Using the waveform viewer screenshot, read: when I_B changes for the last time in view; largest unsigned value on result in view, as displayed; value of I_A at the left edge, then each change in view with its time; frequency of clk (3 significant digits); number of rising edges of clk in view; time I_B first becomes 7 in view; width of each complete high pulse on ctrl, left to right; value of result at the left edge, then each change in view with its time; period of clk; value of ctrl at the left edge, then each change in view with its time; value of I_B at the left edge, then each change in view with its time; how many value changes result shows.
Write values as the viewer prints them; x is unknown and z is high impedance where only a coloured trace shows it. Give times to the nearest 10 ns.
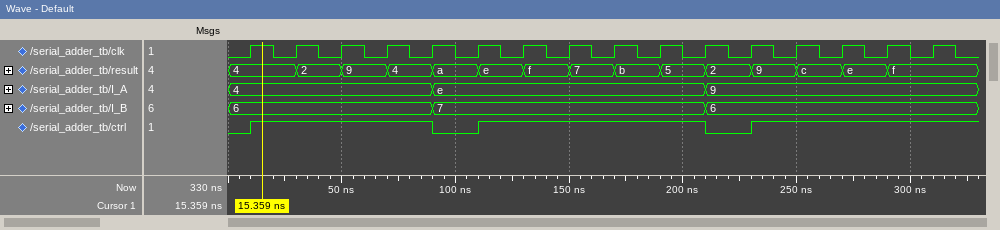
210 ns
f
4, e at 90 ns, 9 at 210 ns
50.0 MHz
16
90 ns
80 ns, 100 ns
4, 2 at 30 ns, 9 at 50 ns, 4 at 70 ns, a at 90 ns, e at 110 ns, f at 130 ns, 7 at 150 ns, b at 170 ns, 5 at 190 ns, 2 at 210 ns, 9 at 230 ns, c at 250 ns, e at 270 ns, f at 290 ns
20 ns
0, 1 at 10 ns, 0 at 90 ns, 1 at 110 ns, 0 at 210 ns, 1 at 230 ns
6, 7 at 90 ns, 6 at 210 ns
14
